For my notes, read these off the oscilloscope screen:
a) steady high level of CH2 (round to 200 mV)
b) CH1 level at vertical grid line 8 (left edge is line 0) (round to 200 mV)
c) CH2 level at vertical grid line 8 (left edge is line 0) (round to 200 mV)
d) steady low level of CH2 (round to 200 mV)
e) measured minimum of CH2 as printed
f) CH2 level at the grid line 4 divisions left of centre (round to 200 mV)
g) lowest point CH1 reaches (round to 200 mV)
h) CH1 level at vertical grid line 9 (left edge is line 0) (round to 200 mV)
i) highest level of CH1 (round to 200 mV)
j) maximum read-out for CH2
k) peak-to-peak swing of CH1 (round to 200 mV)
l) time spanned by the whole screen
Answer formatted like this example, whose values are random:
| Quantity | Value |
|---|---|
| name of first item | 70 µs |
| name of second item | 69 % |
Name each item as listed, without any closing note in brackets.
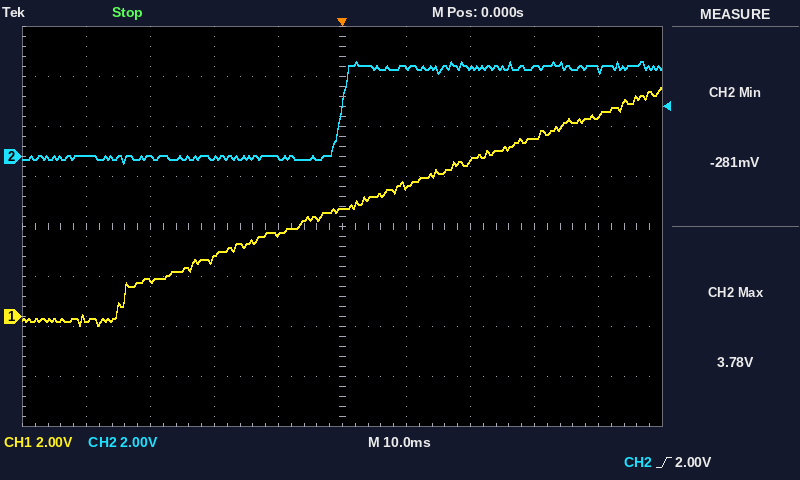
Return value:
| Quantity | Value |
|---|---|
| steady high level of CH2 | 3.6 V |
| CH1 level at vertical grid line 8 (left edge is line 0) | 7.2 V |
| CH2 level at vertical grid line 8 (left edge is line 0) | 3.6 V |
| steady low level of CH2 | 0.0 V |
| measured minimum of CH2 as printed | -281 mV |
| CH2 level at the grid line 4 divisions left of centre | 0.0 V |
| lowest point CH1 reaches | -400 mV |
| CH1 level at vertical grid line 9 (left edge is line 0) | 8.0 V |
| highest level of CH1 | 9.2 V |
| maximum read-out for CH2 | 3.78 V |
| peak-to-peak swing of CH1 | 9.6 V |
| time spanned by the whole screen | 100 ms |
